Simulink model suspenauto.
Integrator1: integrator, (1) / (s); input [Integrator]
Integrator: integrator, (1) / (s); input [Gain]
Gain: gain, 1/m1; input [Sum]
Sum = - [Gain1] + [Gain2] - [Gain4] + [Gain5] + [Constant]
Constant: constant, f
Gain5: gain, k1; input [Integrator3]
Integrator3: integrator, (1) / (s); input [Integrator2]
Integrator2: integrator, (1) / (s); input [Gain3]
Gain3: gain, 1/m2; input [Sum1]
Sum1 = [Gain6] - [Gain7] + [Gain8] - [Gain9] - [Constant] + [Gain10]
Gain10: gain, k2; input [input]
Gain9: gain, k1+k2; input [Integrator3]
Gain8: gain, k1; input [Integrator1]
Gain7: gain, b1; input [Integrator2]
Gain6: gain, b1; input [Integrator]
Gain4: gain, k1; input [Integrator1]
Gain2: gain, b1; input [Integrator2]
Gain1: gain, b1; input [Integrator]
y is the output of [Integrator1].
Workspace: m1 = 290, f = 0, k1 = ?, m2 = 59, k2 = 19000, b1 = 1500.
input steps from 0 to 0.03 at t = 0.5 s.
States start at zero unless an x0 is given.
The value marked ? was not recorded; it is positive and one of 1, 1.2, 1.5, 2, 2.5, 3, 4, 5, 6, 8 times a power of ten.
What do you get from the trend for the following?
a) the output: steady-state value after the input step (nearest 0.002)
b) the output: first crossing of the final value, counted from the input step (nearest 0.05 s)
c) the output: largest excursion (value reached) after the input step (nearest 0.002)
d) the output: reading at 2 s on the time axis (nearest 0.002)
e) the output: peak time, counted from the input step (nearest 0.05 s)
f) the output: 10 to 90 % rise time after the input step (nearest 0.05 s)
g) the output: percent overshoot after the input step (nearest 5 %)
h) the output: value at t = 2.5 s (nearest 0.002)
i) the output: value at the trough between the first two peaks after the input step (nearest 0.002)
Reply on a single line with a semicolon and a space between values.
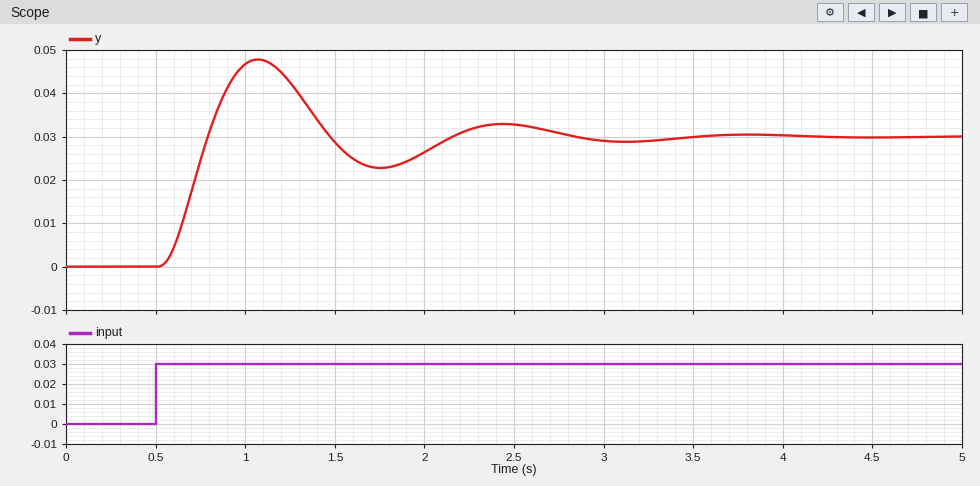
0.030; 0.30 s; 0.048; 0.026; 0.55 s; 0.20 s; 60 %; 0.032; 0.022
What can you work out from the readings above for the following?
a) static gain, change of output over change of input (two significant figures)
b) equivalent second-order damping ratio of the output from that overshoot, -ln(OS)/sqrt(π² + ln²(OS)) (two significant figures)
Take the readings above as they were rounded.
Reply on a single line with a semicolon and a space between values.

1.0; 0.16
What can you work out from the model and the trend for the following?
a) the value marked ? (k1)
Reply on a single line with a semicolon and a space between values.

8000
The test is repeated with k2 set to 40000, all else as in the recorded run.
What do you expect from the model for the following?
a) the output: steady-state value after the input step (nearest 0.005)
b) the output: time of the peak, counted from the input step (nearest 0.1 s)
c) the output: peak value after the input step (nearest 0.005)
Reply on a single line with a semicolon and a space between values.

0.030; 0.5 s; 0.045
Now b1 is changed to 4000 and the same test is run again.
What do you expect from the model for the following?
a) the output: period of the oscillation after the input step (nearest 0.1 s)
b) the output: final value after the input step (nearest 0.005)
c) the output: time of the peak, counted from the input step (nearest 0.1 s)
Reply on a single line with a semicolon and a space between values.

0.9 s; 0.030; 0.5 s
